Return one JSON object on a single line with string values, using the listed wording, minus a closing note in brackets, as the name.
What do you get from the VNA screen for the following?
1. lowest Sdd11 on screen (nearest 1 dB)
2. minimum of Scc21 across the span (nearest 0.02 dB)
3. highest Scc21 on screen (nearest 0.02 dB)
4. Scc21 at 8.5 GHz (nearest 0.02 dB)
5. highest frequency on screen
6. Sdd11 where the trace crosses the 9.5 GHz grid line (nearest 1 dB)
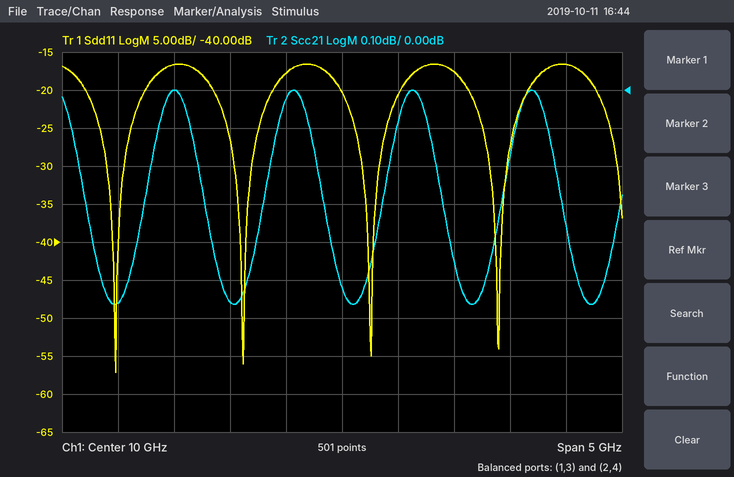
{"lowest Sdd11 on screen": "-57 dB", "minimum of Scc21 across the span": "-0.56 dB", "highest Scc21 on screen": "0.00 dB", "Scc21 at 8.5 GHz": "0.00 dB", "highest frequency on screen": "12.5 GHz", "Sdd11 where the trace crosses the 9.5 GHz grid line": "-18 dB"}
